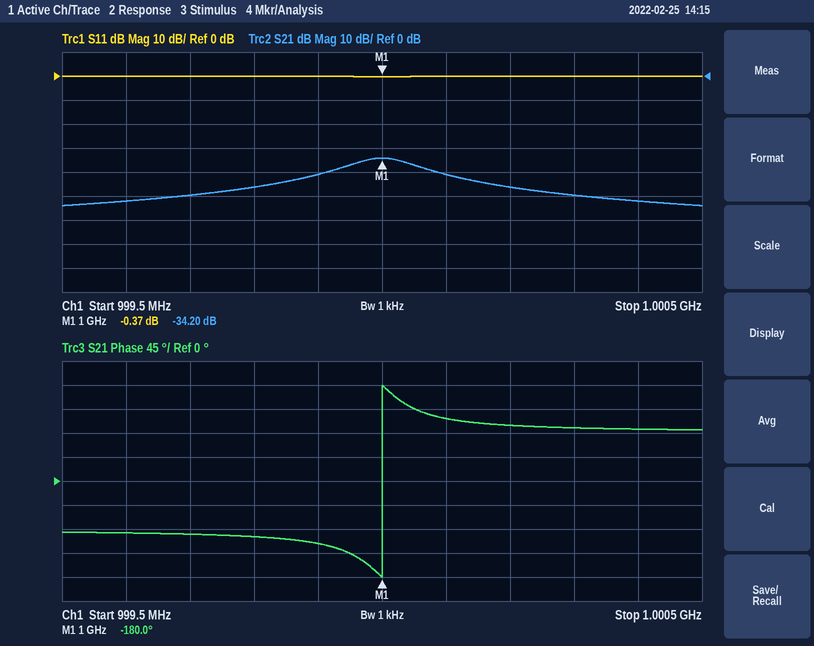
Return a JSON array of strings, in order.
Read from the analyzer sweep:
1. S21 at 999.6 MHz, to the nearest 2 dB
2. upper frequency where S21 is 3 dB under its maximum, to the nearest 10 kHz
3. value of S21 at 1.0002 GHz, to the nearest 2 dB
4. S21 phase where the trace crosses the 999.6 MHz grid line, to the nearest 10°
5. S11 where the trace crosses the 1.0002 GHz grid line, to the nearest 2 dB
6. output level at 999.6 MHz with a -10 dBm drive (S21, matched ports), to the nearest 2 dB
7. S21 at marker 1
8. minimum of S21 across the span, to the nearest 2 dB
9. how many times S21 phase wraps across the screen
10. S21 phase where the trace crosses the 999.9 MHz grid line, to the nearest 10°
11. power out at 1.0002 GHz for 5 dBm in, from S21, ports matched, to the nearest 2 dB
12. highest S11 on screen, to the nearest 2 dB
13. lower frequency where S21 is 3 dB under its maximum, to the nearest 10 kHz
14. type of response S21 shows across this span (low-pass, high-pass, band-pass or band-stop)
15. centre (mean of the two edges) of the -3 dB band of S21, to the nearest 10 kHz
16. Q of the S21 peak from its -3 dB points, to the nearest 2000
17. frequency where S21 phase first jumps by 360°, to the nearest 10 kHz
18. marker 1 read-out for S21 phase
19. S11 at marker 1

["-52 dB", "1.00005 GHz", "-46 dB", "-100°", "0 dB", "-62 dBm", "-34.20 dB", "-54 dB", "1", "-120°", "-42 dBm", "0 dB", "999.95 MHz", "band-pass", "1.00000 GHz", "10000", "1.00000 GHz", "-180.0°", "-0.37 dB"]
